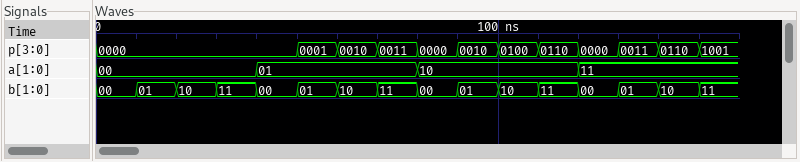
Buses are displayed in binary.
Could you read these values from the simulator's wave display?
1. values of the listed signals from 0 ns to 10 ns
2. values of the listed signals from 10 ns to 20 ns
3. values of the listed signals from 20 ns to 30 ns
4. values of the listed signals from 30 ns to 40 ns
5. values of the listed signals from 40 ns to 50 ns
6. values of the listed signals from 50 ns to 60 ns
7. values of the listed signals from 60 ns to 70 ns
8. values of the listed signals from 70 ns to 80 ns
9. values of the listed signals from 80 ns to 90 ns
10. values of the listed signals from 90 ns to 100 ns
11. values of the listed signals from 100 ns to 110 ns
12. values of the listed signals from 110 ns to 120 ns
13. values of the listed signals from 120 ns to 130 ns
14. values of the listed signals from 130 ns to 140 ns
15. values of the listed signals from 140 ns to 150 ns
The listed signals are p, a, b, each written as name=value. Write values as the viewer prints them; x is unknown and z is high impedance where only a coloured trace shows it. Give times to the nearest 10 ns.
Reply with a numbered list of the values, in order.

1. p=0000, a=00, b=00
2. p=0000, a=00, b=01
3. p=0000, a=00, b=10
4. p=0000, a=00, b=11
5. p=0000, a=01, b=00
6. p=0001, a=01, b=01
7. p=0010, a=01, b=10
8. p=0011, a=01, b=11
9. p=0000, a=10, b=00
10. p=0010, a=10, b=01
11. p=0100, a=10, b=10
12. p=0110, a=10, b=11
13. p=0000, a=11, b=00
14. p=0011, a=11, b=01
15. p=0110, a=11, b=10
